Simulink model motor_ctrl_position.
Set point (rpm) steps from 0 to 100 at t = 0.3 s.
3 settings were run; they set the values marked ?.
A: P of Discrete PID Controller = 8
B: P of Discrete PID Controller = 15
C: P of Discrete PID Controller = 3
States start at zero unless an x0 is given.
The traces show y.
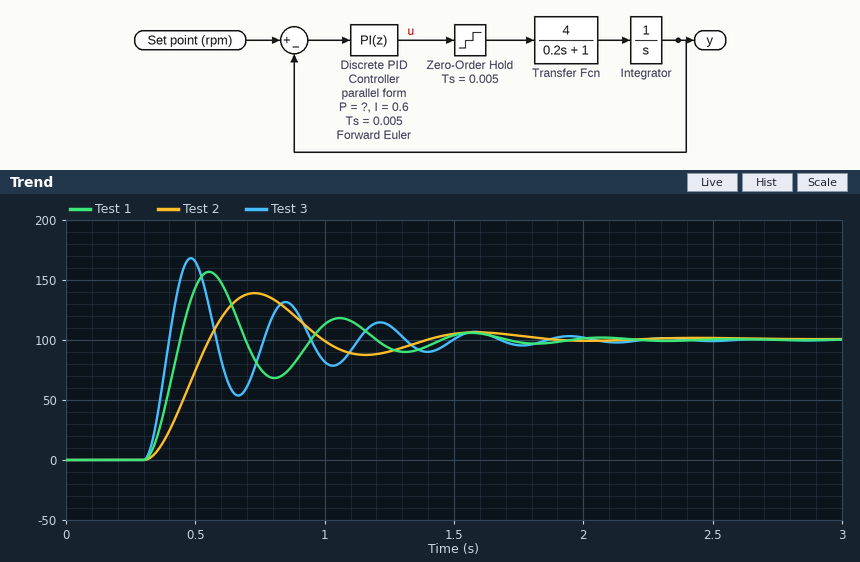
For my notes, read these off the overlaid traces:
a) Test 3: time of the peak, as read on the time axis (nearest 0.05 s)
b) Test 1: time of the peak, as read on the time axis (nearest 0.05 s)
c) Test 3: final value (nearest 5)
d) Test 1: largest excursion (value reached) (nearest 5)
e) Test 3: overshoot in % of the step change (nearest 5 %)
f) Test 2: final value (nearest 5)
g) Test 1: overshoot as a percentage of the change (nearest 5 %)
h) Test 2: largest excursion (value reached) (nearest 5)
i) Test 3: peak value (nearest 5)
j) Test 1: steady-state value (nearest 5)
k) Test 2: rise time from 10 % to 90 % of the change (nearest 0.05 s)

0.50 s
0.55 s
100
155
70 %
100
55 %
140
170
100
0.15 s
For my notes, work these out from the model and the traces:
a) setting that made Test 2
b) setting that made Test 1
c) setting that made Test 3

C
A
B
